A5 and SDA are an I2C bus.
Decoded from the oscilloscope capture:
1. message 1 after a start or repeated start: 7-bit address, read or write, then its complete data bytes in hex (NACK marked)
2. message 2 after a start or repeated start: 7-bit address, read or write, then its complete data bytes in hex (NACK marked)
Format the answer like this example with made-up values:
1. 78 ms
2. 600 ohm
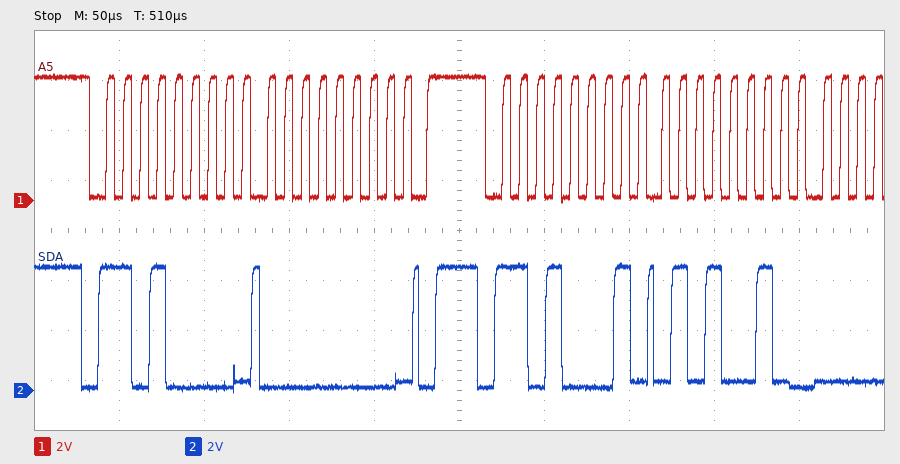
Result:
1. 0x68 write: 00
2. 0x68 read: 52
